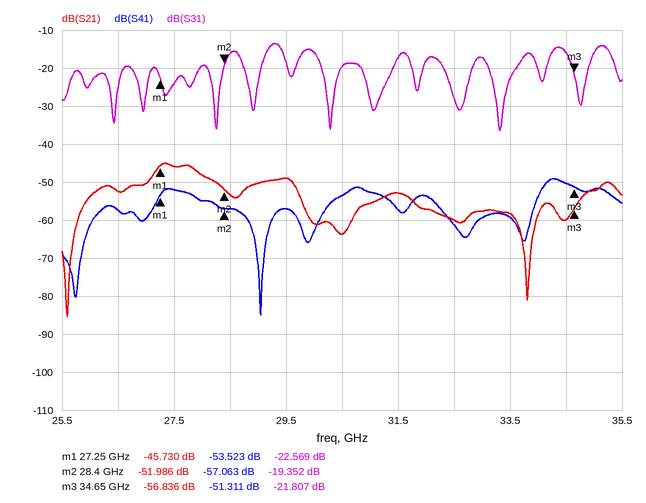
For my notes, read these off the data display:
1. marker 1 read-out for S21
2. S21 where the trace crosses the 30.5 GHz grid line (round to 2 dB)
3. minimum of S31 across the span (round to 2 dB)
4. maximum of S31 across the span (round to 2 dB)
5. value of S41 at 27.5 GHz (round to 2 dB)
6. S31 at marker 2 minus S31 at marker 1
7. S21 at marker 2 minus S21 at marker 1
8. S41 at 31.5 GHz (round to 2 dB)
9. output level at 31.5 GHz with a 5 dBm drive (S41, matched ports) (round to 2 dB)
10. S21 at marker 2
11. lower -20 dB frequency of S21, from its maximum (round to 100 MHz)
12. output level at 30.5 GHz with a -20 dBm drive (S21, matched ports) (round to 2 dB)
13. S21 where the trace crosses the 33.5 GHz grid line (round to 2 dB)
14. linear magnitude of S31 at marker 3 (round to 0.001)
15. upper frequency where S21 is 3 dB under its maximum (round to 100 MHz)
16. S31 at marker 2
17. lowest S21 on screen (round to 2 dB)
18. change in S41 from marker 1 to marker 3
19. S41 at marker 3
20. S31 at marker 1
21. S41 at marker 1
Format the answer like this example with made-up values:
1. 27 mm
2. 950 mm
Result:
1. -45.730 dB
2. -64 dB
3. -36 dB
4. -14 dB
5. -52 dB
6. 3.217 dB
7. -6.256 dB
8. -58 dB
9. -52 dBm
10. -51.986 dB
11. 25.7 GHz
12. -84 dBm
13. -58 dB
14. 0.081
15. 28.0 GHz
16. -19.352 dB
17. -86 dB
18. 2.212 dB
19. -51.311 dB
20. -22.569 dB
21. -53.523 dB
